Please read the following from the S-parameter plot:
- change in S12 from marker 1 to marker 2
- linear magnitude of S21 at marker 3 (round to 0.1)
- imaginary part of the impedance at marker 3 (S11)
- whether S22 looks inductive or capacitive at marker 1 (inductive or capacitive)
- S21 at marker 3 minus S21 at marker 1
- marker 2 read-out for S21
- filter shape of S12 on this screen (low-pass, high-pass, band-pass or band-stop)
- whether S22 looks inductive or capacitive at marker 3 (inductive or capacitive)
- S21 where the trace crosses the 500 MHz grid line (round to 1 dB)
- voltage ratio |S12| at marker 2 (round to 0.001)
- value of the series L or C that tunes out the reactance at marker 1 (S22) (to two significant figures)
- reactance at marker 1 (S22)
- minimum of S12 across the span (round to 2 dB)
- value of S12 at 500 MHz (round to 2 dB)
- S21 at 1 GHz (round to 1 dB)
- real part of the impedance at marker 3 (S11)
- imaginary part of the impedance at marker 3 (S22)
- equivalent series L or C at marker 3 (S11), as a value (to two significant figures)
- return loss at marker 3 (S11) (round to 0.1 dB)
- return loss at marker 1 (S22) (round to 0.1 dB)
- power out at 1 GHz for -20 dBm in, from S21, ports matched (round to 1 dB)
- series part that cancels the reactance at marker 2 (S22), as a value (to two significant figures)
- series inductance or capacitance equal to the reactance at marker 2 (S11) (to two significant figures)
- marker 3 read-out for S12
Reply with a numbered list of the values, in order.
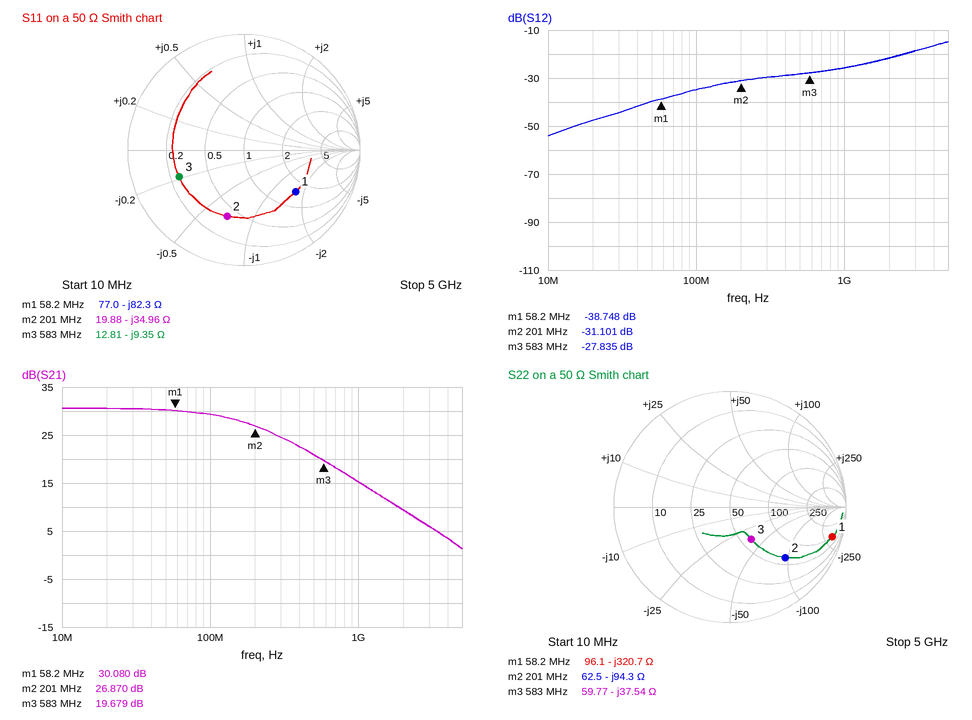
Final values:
1. 7.647 dB
2. 9.6
3. -9.35 Ω
4. capacitive
5. -10.401 dB
6. 26.870 dB
7. high-pass
8. capacitive
9. 21 dB
10. 0.028
11. 880 nH
12. -320.7 Ω
13. -54 dB
14. -28 dB
15. 15 dB
16. 12.81 Ω
17. -37.54 Ω
18. 29 pF
19. 4.4 dB
20. 0.7 dB
21. -5 dBm
22. 75 nH
23. 23 pF
24. -27.835 dB
